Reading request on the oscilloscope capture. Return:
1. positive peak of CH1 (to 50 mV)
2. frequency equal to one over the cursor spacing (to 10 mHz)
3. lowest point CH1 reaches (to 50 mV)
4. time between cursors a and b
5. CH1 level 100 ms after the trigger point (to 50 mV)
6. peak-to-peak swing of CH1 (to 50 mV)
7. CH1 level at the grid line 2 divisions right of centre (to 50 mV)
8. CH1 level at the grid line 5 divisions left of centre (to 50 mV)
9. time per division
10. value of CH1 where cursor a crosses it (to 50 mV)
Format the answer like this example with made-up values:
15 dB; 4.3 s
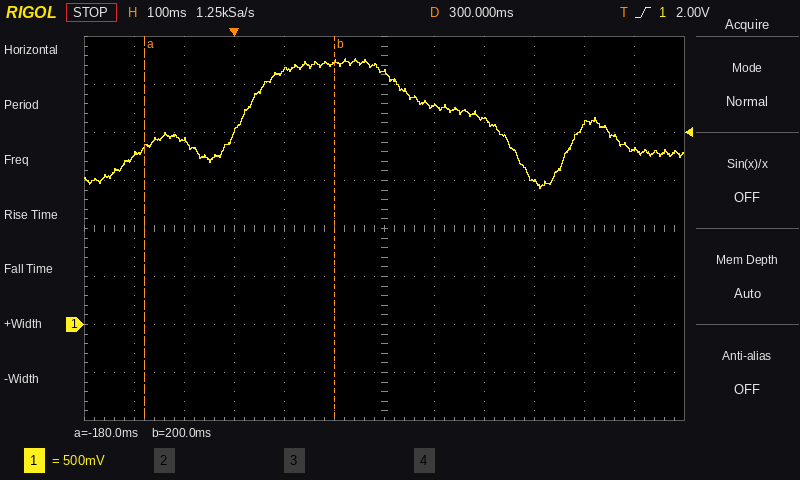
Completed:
2.75 V; 2.63 Hz; 1.40 V; 380 ms; 2.65 V; 1.35 V; 2.15 V; 1.75 V; 100 ms; 1.85 V
